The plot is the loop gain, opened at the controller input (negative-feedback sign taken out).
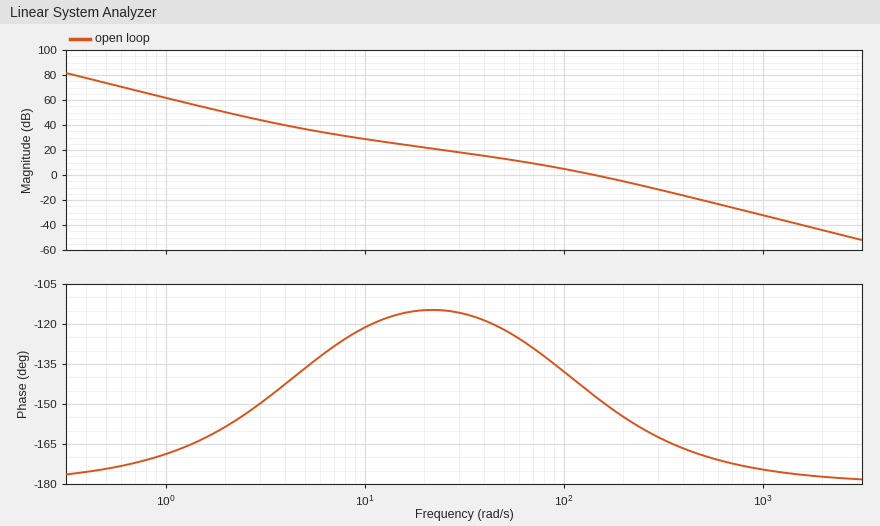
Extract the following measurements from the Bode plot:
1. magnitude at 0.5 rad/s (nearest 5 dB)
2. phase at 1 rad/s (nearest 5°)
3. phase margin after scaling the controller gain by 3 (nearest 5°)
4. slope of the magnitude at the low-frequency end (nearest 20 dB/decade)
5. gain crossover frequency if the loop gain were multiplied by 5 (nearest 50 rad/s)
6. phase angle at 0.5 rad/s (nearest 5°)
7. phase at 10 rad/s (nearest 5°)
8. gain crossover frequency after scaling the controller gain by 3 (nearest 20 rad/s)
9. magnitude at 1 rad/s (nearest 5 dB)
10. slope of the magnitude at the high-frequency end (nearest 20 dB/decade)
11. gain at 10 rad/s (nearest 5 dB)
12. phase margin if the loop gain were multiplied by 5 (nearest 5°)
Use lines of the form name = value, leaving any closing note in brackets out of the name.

magnitude at 0.5 rad/s = 75 dB
phase at 1 rad/s = -170°
phase margin after scaling the controller gain by 3 = 20°
slope of the magnitude at the low-frequency end = -40 dB/decade
gain crossover frequency if the loop gain were multiplied by 5 = 350 rad/s
phase angle at 0.5 rad/s = -175°
phase at 10 rad/s = -120°
gain crossover frequency after scaling the controller gain by 3 = 260 rad/s
magnitude at 1 rad/s = 60 dB
slope of the magnitude at the high-frequency end = -40 dB/decade
gain at 10 rad/s = 30 dB
phase margin if the loop gain were multiplied by 5 = 15°
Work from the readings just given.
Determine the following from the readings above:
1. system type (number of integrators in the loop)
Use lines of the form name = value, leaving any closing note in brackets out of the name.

system type = 2
